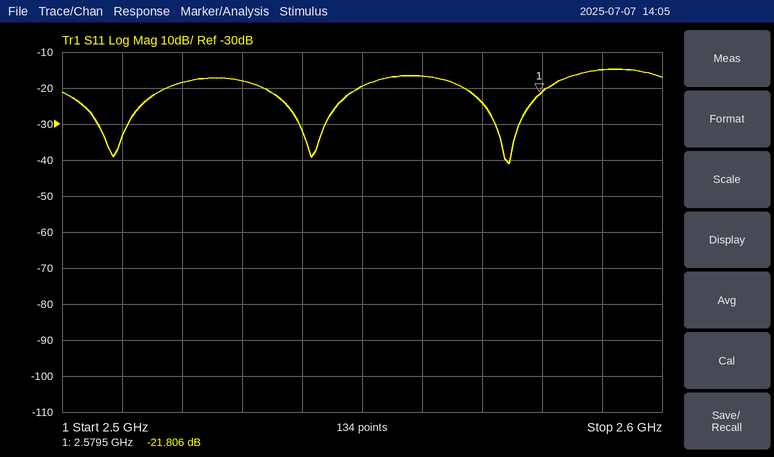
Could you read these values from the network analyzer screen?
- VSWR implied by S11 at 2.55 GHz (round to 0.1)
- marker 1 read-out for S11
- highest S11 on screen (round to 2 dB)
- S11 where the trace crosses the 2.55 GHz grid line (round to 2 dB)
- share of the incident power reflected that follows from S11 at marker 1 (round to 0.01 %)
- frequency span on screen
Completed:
1.2
-21.806 dB
-14 dB
-20 dB
0.66 %
100 MHz
